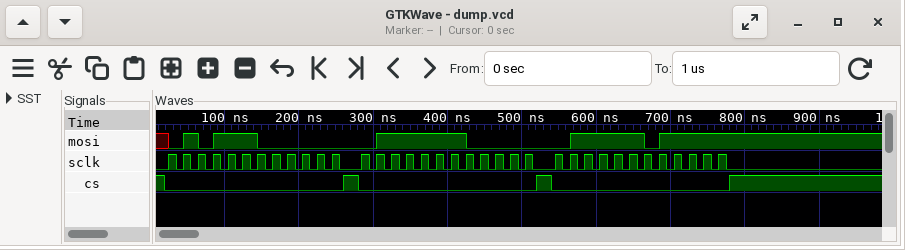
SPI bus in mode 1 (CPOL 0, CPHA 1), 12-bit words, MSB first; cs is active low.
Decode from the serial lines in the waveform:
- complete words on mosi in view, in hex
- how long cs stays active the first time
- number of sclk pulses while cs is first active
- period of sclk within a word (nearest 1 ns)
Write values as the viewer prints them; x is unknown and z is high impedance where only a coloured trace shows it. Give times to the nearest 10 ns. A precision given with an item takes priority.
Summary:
5C0, 7E0, 7DF
240 ns
12
20 ns
